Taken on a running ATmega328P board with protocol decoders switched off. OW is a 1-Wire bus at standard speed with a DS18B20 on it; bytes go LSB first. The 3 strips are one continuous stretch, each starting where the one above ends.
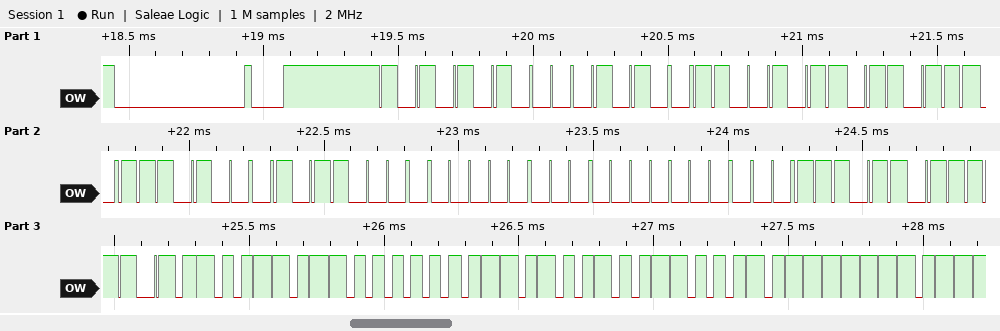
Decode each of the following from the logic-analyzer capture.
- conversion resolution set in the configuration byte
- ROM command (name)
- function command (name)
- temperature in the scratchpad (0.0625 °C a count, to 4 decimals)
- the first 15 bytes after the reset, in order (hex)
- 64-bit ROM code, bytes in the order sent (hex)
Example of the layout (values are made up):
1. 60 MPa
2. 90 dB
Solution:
1. 12 bits
2. Match ROM
3. Read Scratchpad
4. 27.1250 °C
5. 55 28 D3 76 17 0D 00 00 DC BE B2 01 4B 46 7F
6. 28 D3 76 17 0D 00 00 DC
